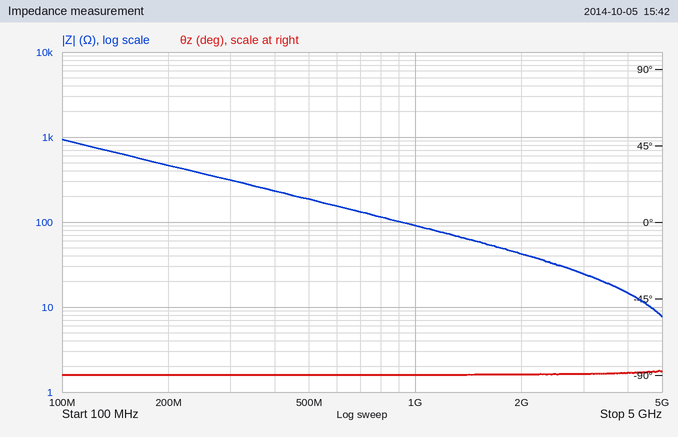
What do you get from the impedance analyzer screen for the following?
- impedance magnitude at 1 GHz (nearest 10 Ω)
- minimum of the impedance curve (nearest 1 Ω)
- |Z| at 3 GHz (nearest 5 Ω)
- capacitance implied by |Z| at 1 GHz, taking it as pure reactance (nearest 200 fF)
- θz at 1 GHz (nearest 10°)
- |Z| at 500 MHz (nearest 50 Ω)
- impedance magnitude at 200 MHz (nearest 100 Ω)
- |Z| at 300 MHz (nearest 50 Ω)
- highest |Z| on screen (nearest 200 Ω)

90 Ω
8 Ω
25 Ω
1.8 pF
-90°
200 Ω
500 Ω
300 Ω
1.0 kΩ
